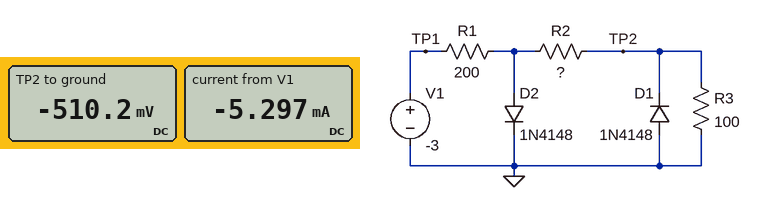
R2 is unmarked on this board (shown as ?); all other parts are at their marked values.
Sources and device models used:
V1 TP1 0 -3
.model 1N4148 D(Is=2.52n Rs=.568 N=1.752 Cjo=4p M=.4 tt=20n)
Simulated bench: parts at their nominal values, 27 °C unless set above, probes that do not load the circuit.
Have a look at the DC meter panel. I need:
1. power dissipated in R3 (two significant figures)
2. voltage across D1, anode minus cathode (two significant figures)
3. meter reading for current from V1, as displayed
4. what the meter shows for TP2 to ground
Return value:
2.6 mW
510 mV
-5.297 mA
-510.2 mV
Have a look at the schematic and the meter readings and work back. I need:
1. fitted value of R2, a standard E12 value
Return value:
270 Ω
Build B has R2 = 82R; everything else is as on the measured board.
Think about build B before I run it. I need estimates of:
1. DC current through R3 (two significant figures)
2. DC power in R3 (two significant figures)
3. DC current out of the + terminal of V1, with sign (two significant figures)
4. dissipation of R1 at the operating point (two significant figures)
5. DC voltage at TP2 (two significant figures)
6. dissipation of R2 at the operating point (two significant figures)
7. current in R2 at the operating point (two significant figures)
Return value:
6.2 mA
3.9 mW
-8.4 mA
14 mW
-620 mV
5.8 mW
8.4 mA
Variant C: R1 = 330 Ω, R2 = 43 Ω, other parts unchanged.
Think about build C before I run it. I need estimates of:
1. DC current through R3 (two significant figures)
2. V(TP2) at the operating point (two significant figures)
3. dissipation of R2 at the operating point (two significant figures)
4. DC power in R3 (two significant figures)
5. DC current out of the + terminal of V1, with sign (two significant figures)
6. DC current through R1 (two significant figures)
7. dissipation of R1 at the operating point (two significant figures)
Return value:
5.7 mA
-570 mV
1.8 mW
3.3 mW
-6.5 mA
6.5 mA
14 mW
